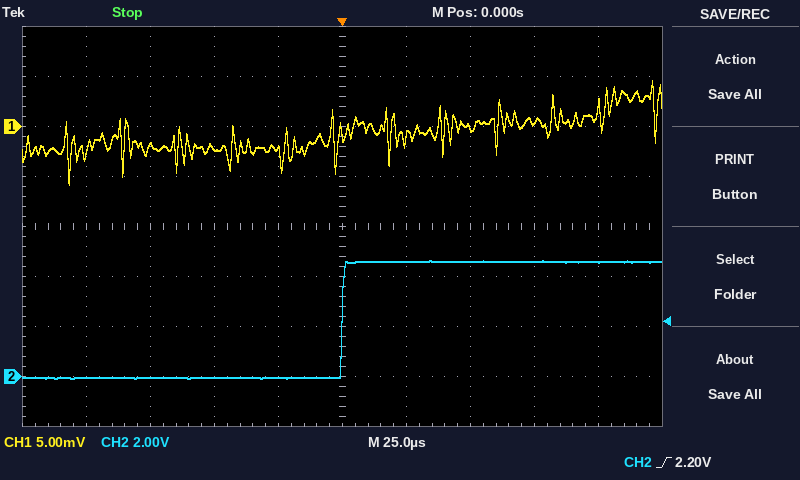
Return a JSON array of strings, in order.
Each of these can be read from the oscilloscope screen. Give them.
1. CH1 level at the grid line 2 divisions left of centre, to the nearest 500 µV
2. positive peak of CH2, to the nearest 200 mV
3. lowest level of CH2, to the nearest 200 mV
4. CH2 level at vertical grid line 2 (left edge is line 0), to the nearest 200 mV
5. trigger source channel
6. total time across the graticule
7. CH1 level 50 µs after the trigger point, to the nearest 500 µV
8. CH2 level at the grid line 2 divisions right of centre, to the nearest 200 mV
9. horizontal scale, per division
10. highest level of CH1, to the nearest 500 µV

["-2.0 mV", "4.6 V", "0.0 V", "0.0 V", "CH2", "250 µs", "0.0 mV", "4.6 V", "25 µs", "4.5 mV"]
